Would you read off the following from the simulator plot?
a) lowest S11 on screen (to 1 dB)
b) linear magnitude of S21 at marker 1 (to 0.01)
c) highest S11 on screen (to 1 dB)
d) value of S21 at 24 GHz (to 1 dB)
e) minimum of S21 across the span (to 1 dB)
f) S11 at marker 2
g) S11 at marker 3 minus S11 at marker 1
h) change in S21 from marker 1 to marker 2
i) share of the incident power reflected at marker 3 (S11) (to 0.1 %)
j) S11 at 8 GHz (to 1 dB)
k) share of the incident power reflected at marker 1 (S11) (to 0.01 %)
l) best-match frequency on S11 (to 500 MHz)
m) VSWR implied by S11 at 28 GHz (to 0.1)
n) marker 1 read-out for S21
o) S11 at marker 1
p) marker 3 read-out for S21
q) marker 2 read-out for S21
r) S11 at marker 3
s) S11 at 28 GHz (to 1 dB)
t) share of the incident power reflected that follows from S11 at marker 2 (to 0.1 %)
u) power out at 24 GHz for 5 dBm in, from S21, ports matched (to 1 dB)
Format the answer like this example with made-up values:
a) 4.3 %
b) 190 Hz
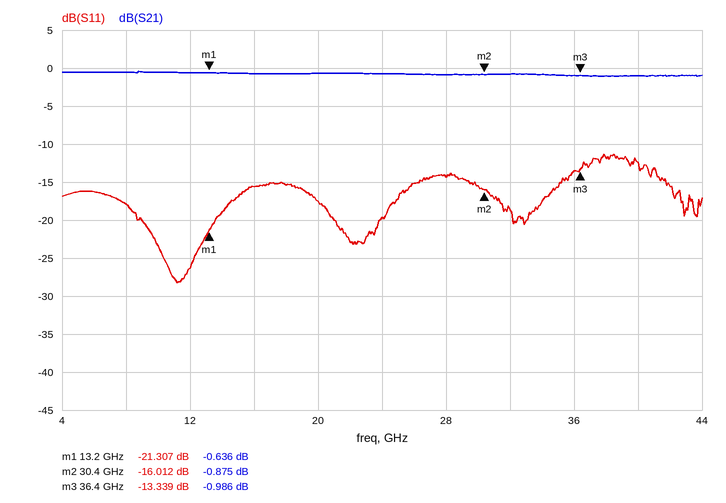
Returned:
a) -28 dB
b) 0.93
c) -11 dB
d) -1 dB
e) -1 dB
f) -16.012 dB
g) 7.968 dB
h) -0.239 dB
i) 4.6 %
j) -18 dB
k) 0.74 %
l) 11.0 GHz
m) 1.5
n) -0.636 dB
o) -21.307 dB
p) -0.986 dB
q) -0.875 dB
r) -13.339 dB
s) -14 dB
t) 2.5 %
u) 4 dBm
